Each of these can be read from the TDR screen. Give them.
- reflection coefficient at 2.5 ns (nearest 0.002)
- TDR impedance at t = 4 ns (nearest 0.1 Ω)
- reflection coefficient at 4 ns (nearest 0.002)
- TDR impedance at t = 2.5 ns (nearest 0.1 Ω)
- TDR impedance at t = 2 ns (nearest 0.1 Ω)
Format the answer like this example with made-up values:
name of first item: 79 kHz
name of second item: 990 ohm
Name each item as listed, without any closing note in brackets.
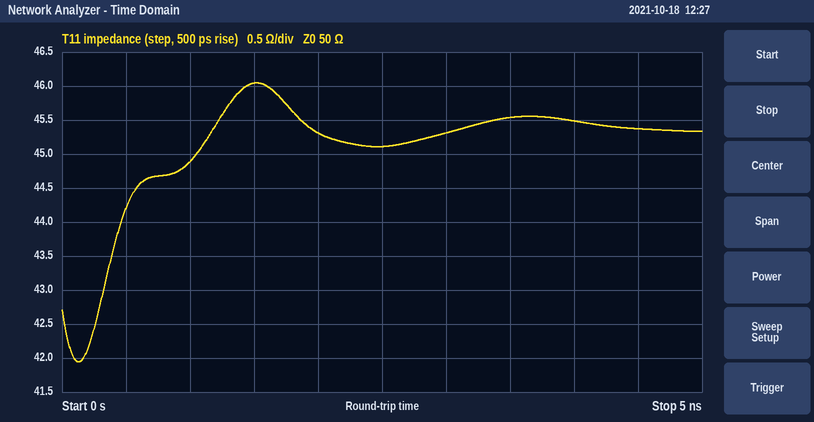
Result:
reflection coefficient at 2.5 ns: -0.052
TDR impedance at t = 4 ns: 45.5 Ω
reflection coefficient at 4 ns: -0.048
TDR impedance at t = 2.5 ns: 45.1 Ω
TDR impedance at t = 2 ns: 45.3 Ω
